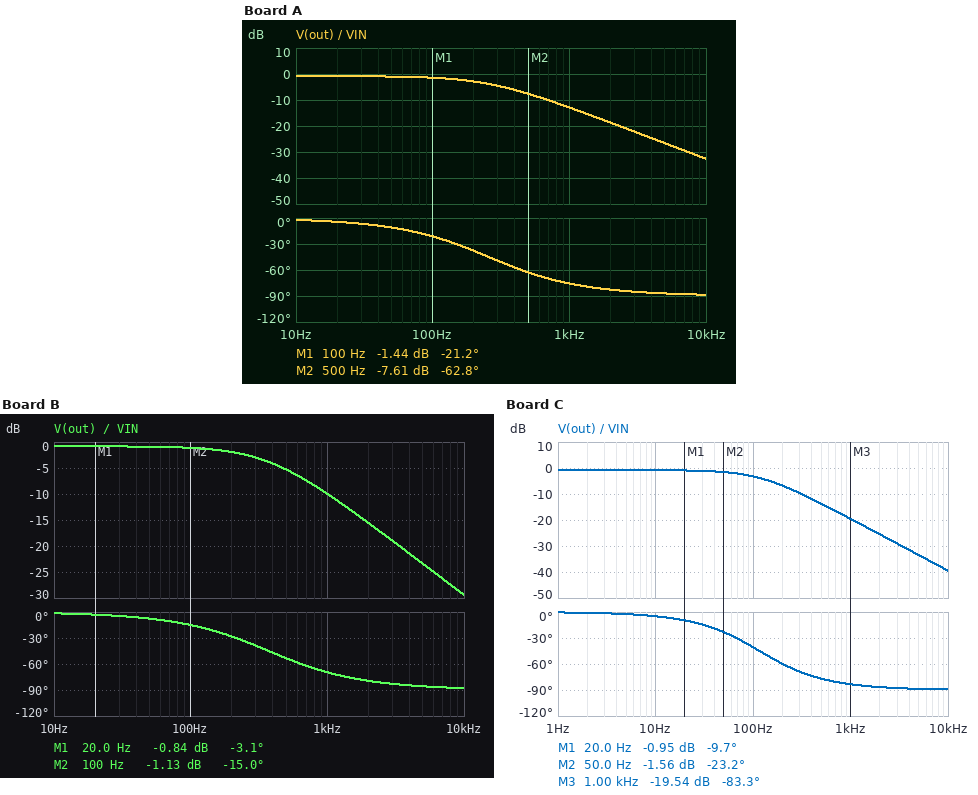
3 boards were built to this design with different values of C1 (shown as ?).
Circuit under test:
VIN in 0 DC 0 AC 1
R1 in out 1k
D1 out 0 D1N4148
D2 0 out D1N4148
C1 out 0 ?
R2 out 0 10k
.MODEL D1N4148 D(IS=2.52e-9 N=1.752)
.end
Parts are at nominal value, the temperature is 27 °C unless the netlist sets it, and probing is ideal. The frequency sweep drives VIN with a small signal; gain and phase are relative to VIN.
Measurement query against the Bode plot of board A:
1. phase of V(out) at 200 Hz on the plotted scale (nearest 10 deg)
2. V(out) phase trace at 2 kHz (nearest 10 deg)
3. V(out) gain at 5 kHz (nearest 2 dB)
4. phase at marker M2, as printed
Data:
-40 deg
-80 deg
-26 dB
-62.8 deg
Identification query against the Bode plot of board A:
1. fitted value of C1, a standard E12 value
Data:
680 nF
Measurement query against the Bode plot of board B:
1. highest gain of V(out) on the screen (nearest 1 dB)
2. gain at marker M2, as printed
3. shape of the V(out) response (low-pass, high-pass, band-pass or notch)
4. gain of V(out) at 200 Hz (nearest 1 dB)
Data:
-1 dB
-1.13 dB
low-pass
-2 dB
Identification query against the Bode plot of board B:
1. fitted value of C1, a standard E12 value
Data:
470 nF
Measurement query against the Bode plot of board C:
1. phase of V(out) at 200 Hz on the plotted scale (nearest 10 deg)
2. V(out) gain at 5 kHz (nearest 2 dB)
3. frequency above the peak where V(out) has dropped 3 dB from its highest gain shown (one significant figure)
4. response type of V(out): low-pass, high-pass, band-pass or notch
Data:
-60 deg
-34 dB
100 Hz
low-pass
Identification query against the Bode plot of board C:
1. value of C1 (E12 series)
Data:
1.5 µF
